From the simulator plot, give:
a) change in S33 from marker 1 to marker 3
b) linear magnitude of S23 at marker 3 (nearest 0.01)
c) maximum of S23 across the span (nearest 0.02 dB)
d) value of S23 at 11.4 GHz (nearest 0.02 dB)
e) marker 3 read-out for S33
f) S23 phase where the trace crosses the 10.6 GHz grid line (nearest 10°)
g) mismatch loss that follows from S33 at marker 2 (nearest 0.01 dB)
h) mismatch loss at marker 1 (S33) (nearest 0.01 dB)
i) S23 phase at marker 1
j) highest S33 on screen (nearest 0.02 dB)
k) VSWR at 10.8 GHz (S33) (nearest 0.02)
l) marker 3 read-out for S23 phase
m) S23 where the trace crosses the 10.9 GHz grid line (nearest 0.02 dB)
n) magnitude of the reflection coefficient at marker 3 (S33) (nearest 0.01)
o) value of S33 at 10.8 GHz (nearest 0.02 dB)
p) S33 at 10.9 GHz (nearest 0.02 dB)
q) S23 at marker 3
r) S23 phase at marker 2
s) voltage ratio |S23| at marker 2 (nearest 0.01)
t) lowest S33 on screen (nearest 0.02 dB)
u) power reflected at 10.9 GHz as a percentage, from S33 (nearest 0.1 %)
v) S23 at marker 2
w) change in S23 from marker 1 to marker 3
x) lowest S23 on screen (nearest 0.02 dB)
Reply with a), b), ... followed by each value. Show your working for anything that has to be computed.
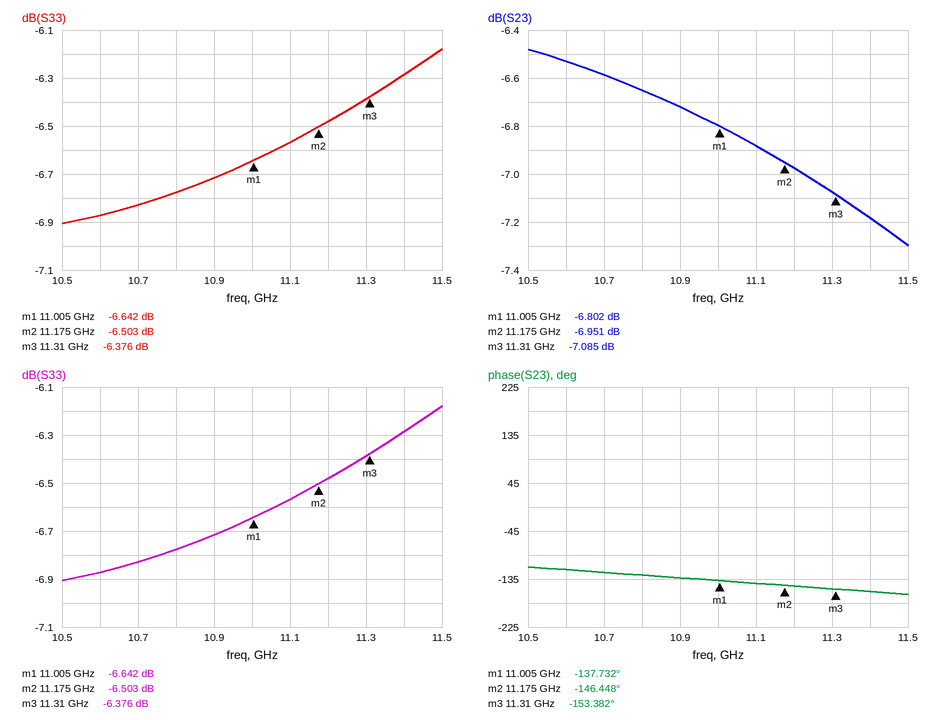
a) -6.376 − (-6.642) = 0.266 dB
b) 10^(-7.085/20) ≈ 0.44
c) -6.48 dB
d) -7.18 dB
e) -6.376 dB
f) -120°
g) −10 log10(1 − 10^(-6.503/10)) ≈ 1.10 dB
h) −10 log10(1 − 10^(-6.642/10)) ≈ 1.06 dB
i) -137.732°
j) -6.18 dB
k) |Γ| = 10^(-6.78/20) = 0.4581; VSWR = (1 + 0.4581)/(1 − 0.4581) ≈ 2.69, so 2.70 to the nearest 0.02
l) -153.382°
m) -6.72 dB
n) 10^(-6.376/20) ≈ 0.48
o) -6.78 dB
p) -6.72 dB
q) -7.085 dB
r) -146.448°
s) 10^(-6.951/20) ≈ 0.45
t) -6.90 dB
u) 10^(-6.72/10) ≈ 21.3 %
v) -6.951 dB
w) -7.085 − (-6.802) = -0.283 dB
x) -7.30 dB
